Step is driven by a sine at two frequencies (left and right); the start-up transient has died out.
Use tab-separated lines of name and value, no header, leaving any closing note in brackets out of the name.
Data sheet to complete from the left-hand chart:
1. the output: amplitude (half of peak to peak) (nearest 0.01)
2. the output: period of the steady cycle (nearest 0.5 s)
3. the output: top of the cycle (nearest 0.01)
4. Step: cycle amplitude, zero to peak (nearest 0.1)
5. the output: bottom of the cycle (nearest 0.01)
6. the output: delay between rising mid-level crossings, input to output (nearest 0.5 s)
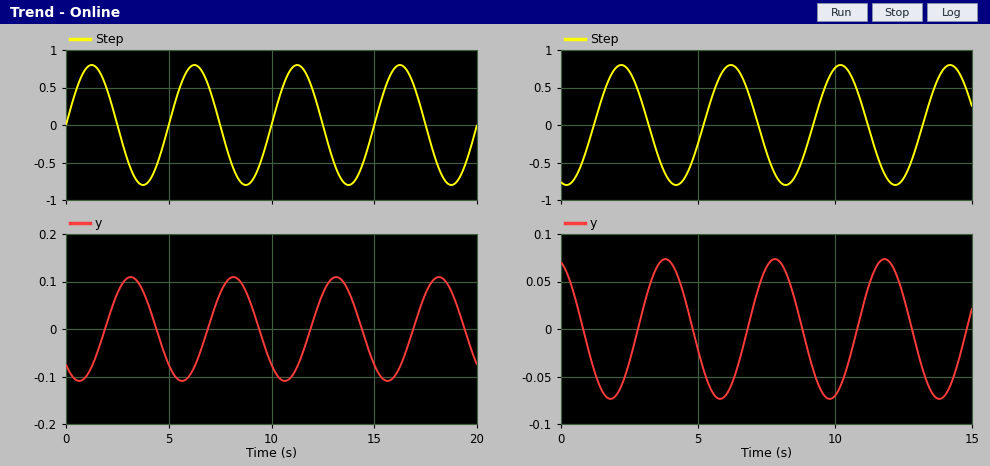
the output: amplitude (half of peak to peak)	0.11
the output: period of the steady cycle	5.0 s
the output: top of the cycle	0.11
Step: cycle amplitude, zero to peak	0.8
the output: bottom of the cycle	-0.11
the output: delay between rising mid-level crossings, input to output	2.0 s
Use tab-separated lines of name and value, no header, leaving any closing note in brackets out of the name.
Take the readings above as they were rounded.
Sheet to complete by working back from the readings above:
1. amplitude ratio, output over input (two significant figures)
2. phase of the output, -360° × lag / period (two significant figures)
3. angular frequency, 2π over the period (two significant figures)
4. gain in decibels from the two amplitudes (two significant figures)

amplitude ratio, output over input	0.14
phase of the output, -360° × lag / period	-140°
angular frequency, 2π over the period	1.3 rad/s
gain in decibels from the two amplitudes	-17 dB
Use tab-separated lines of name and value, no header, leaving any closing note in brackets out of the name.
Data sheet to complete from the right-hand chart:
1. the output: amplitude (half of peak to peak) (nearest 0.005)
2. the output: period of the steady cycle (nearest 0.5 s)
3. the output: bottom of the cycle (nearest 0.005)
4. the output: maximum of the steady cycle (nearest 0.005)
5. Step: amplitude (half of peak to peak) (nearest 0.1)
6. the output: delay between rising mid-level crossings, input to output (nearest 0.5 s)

the output: amplitude (half of peak to peak)	0.075
the output: period of the steady cycle	4.0 s
the output: bottom of the cycle	-0.075
the output: maximum of the steady cycle	0.075
Step: amplitude (half of peak to peak)	0.8
the output: delay between rising mid-level crossings, input to output	1.5 s
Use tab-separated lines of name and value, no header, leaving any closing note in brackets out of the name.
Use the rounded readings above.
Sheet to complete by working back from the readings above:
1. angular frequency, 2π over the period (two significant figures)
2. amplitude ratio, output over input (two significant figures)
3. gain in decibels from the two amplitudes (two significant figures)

angular frequency, 2π over the period	1.6 rad/s
amplitude ratio, output over input	0.094
gain in decibels from the two amplitudes	-21 dB
